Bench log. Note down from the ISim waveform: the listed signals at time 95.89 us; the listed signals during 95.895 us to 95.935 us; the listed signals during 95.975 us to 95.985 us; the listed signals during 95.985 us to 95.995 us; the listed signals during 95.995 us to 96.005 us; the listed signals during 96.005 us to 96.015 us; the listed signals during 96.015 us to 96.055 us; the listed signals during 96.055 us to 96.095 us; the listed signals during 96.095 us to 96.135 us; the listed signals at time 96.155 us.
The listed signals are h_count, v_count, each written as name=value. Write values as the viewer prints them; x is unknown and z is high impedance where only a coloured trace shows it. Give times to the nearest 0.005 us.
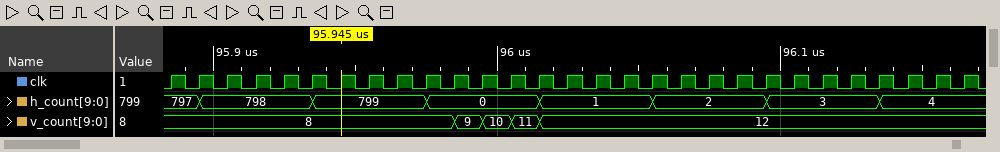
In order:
h_count=797, v_count=8
h_count=798, v_count=8
h_count=0, v_count=8
h_count=0, v_count=9
h_count=0, v_count=10
h_count=0, v_count=11
h_count=1, v_count=12
h_count=2, v_count=12
h_count=3, v_count=12
h_count=4, v_count=12
